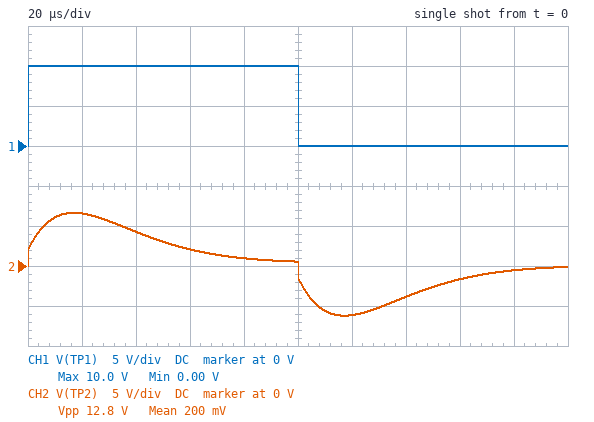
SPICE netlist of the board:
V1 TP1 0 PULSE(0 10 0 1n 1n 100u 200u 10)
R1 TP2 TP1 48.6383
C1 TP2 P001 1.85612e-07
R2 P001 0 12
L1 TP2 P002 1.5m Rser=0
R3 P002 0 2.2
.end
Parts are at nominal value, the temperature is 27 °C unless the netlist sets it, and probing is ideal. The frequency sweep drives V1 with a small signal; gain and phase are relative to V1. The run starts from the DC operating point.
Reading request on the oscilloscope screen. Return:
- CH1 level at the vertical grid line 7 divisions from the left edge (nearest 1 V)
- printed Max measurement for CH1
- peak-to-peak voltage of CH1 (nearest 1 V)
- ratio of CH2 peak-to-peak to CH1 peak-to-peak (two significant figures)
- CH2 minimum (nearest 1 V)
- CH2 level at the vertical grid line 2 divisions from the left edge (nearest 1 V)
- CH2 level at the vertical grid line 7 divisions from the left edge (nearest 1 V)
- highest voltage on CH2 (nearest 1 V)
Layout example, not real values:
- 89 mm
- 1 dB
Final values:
- 0 V
- 10.0 V
- 10 V
- 1.3
- -6 V
- 4 V
- -4 V
- 7 V
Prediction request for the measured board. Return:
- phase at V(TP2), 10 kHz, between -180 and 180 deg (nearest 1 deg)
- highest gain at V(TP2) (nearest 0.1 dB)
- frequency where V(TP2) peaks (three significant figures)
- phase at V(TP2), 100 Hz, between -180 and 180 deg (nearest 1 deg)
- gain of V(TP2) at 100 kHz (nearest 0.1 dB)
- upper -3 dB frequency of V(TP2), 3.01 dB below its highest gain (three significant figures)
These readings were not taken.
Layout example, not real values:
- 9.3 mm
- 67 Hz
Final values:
- -2 deg
- -0.7 dB
- 8.83 kHz
- 22 deg
- -12.3 dB
- 20.1 kHz
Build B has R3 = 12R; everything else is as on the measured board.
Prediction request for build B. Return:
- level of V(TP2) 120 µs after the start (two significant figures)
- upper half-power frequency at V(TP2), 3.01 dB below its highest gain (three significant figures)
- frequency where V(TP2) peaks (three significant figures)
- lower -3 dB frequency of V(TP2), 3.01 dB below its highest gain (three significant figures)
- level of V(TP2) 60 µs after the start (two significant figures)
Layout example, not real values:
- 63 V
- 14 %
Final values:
- -4.7 V
- 21.6 kHz
- 9.54 kHz
- 4.22 kHz
- 3.0 V
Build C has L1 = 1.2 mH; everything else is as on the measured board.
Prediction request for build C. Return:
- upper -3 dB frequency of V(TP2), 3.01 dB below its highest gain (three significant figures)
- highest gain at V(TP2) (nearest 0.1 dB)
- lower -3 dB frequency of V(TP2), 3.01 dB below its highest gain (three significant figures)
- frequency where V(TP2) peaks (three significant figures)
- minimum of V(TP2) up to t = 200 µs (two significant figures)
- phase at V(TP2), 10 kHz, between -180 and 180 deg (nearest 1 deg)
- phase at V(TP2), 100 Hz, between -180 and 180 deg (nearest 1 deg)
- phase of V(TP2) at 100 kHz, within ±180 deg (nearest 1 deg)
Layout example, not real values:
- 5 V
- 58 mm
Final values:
- 21.2 kHz
- -0.8 dB
- 4.71 kHz
- 9.88 kHz
- -6.0 V
- 5 deg
- 18 deg
- -27 deg
